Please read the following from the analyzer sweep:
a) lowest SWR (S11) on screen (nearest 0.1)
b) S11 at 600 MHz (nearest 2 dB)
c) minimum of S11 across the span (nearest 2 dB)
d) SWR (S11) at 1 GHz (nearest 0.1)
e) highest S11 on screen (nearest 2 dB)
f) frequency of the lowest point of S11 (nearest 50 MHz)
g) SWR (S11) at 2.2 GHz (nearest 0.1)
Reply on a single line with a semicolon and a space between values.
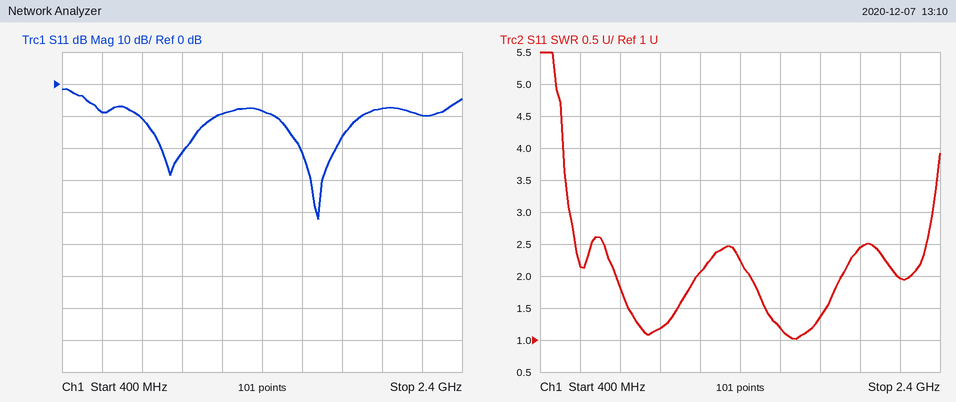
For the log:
1.0; -8 dB; -42 dB; 1.2; -2 dB; 1.70 GHz; 2.0
